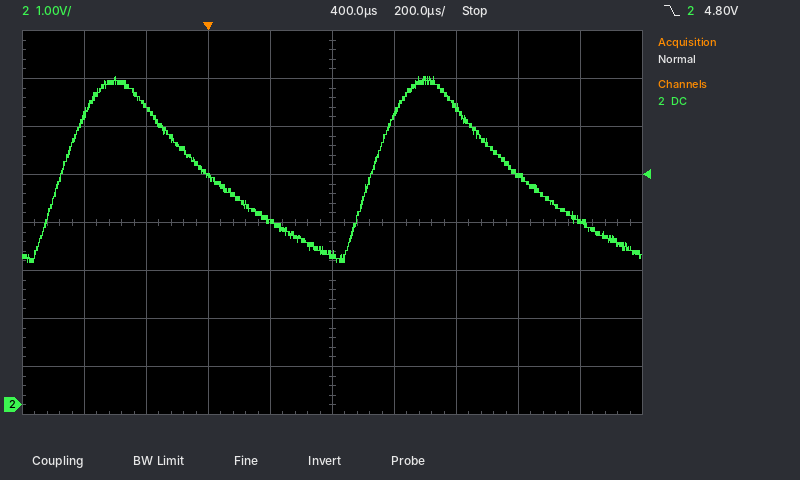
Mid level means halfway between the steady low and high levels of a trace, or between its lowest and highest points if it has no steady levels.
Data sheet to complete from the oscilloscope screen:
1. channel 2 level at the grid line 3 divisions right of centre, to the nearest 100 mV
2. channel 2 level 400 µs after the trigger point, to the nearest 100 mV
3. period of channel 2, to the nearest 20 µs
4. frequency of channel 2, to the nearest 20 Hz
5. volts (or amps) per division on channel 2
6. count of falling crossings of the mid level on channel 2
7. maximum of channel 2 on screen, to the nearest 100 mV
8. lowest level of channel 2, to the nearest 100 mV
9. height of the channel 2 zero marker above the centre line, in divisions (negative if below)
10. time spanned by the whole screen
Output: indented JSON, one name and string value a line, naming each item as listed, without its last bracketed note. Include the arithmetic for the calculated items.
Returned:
{
  "channel 2 level at the grid line 3 divisions right of centre, to the nearest 100 mV": "4.8 V",
  "channel 2 level 400 µs after the trigger point, to the nearest 100 mV": "3.1 V",
  "period of channel 2, to the nearest 20 µs": "1.00 ms",
  "frequency of channel 2, to the nearest 20 Hz": "1 / 1.00 ms ≈ 1.00 kHz",
  "volts (or amps) per division on channel 2": "1 V",
  "count of falling crossings of the mid level on channel 2": "2",
  "maximum of channel 2 on screen, to the nearest 100 mV": "6.8 V",
  "lowest level of channel 2, to the nearest 100 mV": "3.0 V",
  "height of the channel 2 zero marker above the centre line, in divisions": "-3.8 div",
  "time spanned by the whole screen": "2 ms"
}
